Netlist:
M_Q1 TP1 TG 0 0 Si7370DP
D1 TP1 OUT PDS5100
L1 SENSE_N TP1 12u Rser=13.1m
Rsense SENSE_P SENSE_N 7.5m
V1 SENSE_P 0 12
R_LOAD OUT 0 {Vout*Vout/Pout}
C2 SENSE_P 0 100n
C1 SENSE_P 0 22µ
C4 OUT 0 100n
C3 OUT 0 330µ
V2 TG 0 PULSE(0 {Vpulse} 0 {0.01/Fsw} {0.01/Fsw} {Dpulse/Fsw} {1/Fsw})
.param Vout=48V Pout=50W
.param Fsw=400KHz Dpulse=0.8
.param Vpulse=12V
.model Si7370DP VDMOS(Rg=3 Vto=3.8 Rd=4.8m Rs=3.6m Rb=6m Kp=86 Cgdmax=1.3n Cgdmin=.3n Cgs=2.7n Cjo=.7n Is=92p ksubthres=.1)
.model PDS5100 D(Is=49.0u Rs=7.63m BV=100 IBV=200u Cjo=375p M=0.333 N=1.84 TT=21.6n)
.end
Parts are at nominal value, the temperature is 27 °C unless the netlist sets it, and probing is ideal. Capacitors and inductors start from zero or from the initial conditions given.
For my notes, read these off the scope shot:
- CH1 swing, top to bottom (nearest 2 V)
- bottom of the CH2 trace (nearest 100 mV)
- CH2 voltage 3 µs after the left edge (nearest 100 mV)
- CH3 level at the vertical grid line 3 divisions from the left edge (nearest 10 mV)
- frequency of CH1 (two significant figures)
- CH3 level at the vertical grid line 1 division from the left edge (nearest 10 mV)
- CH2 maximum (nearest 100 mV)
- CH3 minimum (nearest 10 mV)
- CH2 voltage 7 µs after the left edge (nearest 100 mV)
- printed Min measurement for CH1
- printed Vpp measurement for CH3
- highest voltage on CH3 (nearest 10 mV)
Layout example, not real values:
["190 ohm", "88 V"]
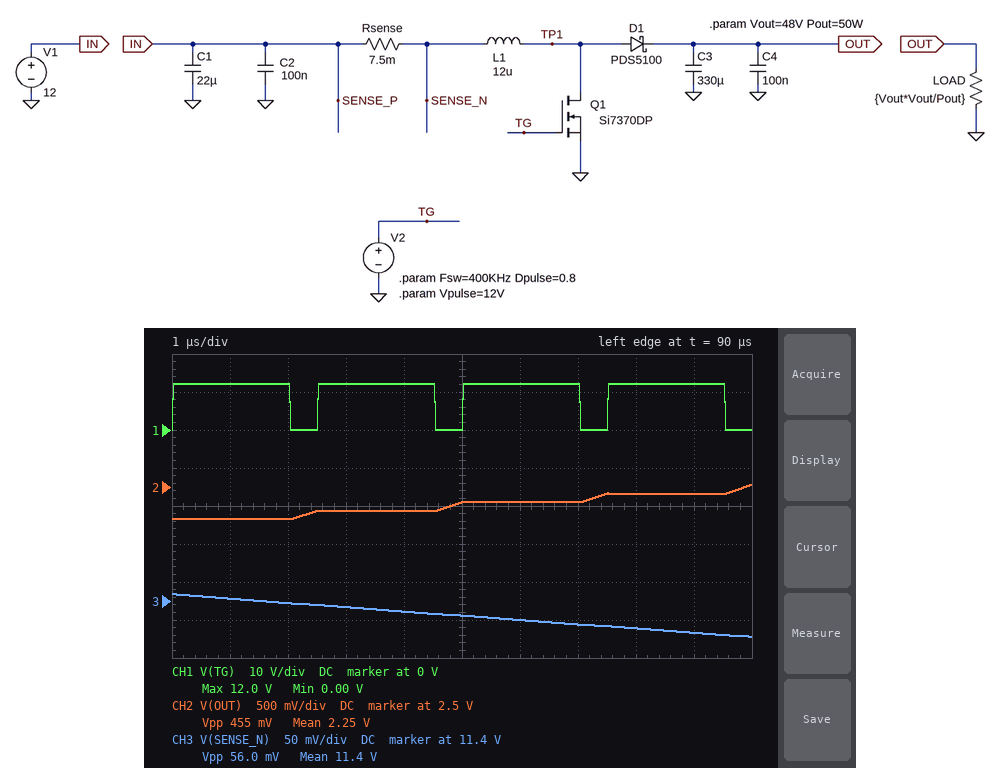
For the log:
["12 V", "2.1 V", "2.2 V", "11.39 V", "400 kHz", "11.40 V", "2.5 V", "11.35 V", "2.3 V", "0.00 V", "56.0 mV", "11.41 V"]
